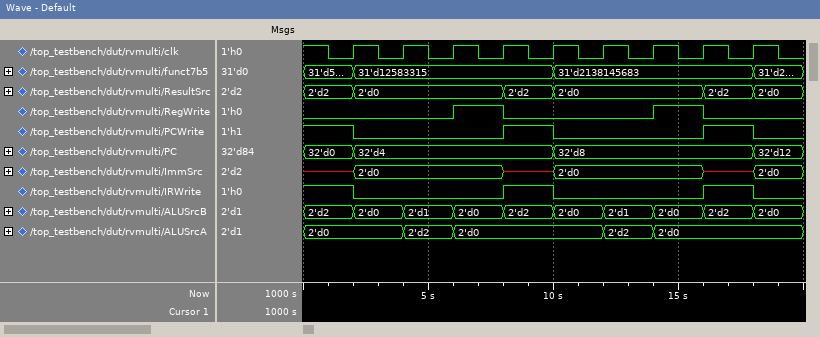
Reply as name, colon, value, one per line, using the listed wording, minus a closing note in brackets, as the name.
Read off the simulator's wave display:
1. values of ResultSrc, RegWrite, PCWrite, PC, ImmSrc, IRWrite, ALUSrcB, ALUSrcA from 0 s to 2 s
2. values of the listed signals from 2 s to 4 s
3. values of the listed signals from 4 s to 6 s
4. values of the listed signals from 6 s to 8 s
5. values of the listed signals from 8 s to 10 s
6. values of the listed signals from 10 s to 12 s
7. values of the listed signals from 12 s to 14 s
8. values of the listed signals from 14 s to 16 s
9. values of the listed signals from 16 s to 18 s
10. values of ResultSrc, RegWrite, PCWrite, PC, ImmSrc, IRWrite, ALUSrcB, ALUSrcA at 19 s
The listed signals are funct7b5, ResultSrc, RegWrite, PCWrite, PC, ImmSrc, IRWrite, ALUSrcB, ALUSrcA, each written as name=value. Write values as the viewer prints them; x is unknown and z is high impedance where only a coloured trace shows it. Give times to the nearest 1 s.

values of ResultSrc, RegWrite, PCWrite, PC, ImmSrc, IRWrite, ALUSrcB, ALUSrcA from 0 s to 2 s: ResultSrc=2'd2, RegWrite=0, PCWrite=1, PC=32'd0, ImmSrc=x, IRWrite=1, ALUSrcB=2'd2, ALUSrcA=2'd0
values of the listed signals from 2 s to 4 s: funct7b5=31'd12583315, ResultSrc=2'd0, RegWrite=0, PCWrite=0, PC=32'd4, ImmSrc=2'd0, IRWrite=0, ALUSrcB=2'd0, ALUSrcA=2'd0
values of the listed signals from 4 s to 6 s: funct7b5=31'd12583315, ResultSrc=2'd0, RegWrite=0, PCWrite=0, PC=32'd4, ImmSrc=2'd0, IRWrite=0, ALUSrcB=2'd1, ALUSrcA=2'd2
values of the listed signals from 6 s to 8 s: funct7b5=31'd12583315, ResultSrc=2'd0, RegWrite=1, PCWrite=0, PC=32'd4, ImmSrc=2'd0, IRWrite=0, ALUSrcB=2'd0, ALUSrcA=2'd0
values of the listed signals from 8 s to 10 s: funct7b5=31'd12583315, ResultSrc=2'd2, RegWrite=0, PCWrite=1, PC=32'd4, ImmSrc=x, IRWrite=1, ALUSrcB=2'd2, ALUSrcA=2'd0
values of the listed signals from 10 s to 12 s: funct7b5=31'd2138145683, ResultSrc=2'd0, RegWrite=0, PCWrite=0, PC=32'd8, ImmSrc=2'd0, IRWrite=0, ALUSrcB=2'd0, ALUSrcA=2'd0
values of the listed signals from 12 s to 14 s: funct7b5=31'd2138145683, ResultSrc=2'd0, RegWrite=0, PCWrite=0, PC=32'd8, ImmSrc=2'd0, IRWrite=0, ALUSrcB=2'd1, ALUSrcA=2'd2
values of the listed signals from 14 s to 16 s: funct7b5=31'd2138145683, ResultSrc=2'd0, RegWrite=1, PCWrite=0, PC=32'd8, ImmSrc=2'd0, IRWrite=0, ALUSrcB=2'd0, ALUSrcA=2'd0
values of the listed signals from 16 s to 18 s: funct7b5=31'd2138145683, ResultSrc=2'd2, RegWrite=0, PCWrite=1, PC=32'd8, ImmSrc=x, IRWrite=1, ALUSrcB=2'd2, ALUSrcA=2'd0
values of ResultSrc, RegWrite, PCWrite, PC, ImmSrc, IRWrite, ALUSrcB, ALUSrcA at 19 s: ResultSrc=2'd0, RegWrite=0, PCWrite=0, PC=32'd12, ImmSrc=2'd0, IRWrite=0, ALUSrcB=2'd0, ALUSrcA=2'd0
